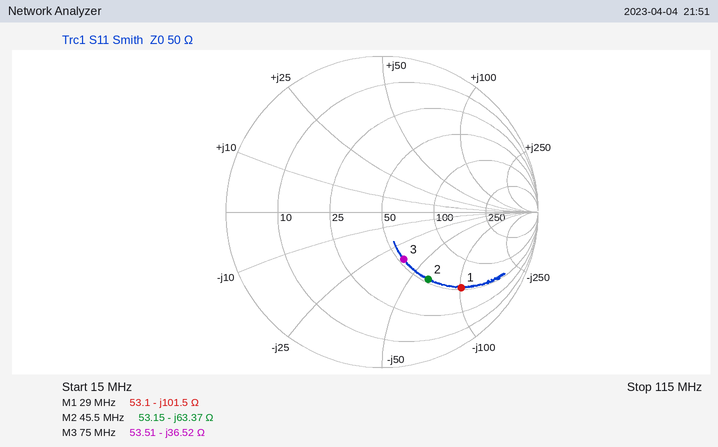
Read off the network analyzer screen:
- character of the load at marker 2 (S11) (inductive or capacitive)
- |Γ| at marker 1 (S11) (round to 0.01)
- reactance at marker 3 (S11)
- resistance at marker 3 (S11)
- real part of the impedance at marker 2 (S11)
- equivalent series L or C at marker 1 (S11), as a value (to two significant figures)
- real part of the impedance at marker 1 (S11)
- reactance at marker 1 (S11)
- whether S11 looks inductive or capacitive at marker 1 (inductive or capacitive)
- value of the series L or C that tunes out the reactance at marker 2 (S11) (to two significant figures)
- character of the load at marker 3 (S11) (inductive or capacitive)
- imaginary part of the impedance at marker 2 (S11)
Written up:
capacitive
0.70
-36.52 Ω
53.51 Ω
53.15 Ω
54 pF
53.1 Ω
-101.5 Ω
capacitive
220 nH
capacitive
-63.37 Ω
